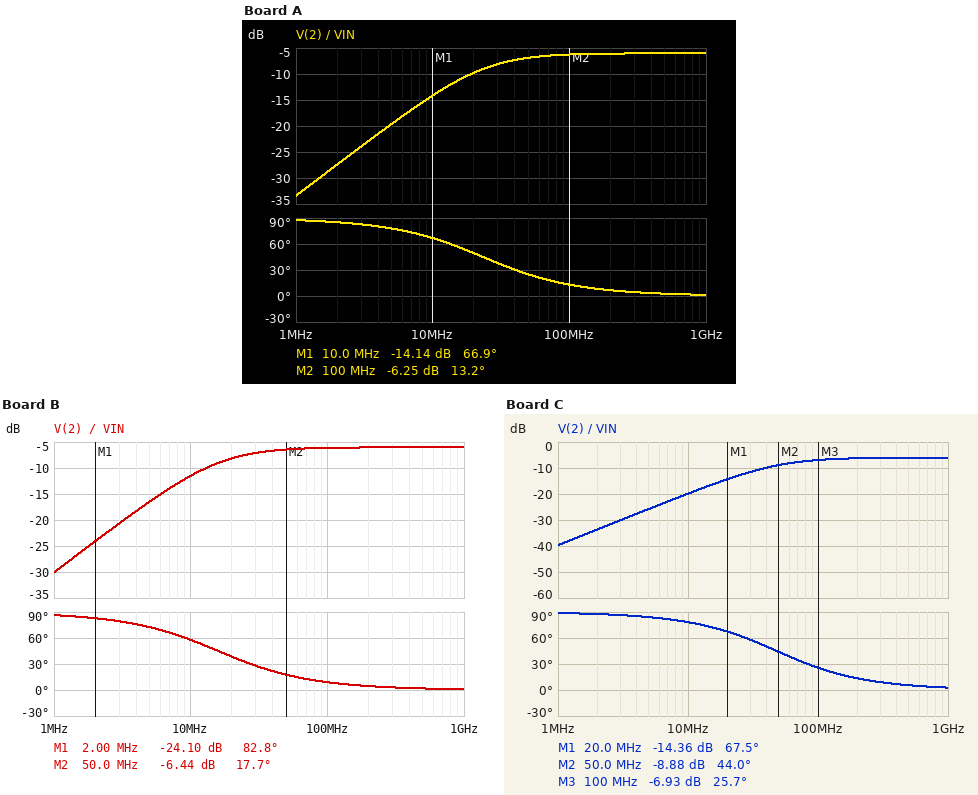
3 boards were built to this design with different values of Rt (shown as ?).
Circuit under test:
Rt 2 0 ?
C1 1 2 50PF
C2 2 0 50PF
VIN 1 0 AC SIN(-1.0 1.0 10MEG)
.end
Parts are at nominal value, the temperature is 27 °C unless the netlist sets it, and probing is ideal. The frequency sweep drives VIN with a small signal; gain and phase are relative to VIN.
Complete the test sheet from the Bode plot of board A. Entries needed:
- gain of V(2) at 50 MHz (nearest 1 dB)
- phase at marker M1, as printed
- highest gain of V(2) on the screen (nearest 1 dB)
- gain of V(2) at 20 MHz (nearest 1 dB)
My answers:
-7 dB
66.9 deg
-6 dB
-10 dB
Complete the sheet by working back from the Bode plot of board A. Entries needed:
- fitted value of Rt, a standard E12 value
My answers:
68 Ω
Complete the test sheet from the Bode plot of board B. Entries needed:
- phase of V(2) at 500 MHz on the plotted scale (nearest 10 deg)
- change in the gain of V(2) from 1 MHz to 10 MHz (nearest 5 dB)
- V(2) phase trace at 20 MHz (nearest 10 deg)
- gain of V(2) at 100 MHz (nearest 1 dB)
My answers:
0 deg
20 dB
40 deg
-6 dB
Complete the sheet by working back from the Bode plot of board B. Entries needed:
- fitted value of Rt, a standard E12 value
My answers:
100 Ω
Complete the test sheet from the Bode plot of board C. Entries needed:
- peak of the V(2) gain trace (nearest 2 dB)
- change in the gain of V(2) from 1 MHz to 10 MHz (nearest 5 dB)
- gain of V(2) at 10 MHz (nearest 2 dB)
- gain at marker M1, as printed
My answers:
-6 dB
20 dB
-20 dB
-14.36 dB
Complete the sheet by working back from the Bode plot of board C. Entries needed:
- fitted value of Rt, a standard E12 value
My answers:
33 Ω
